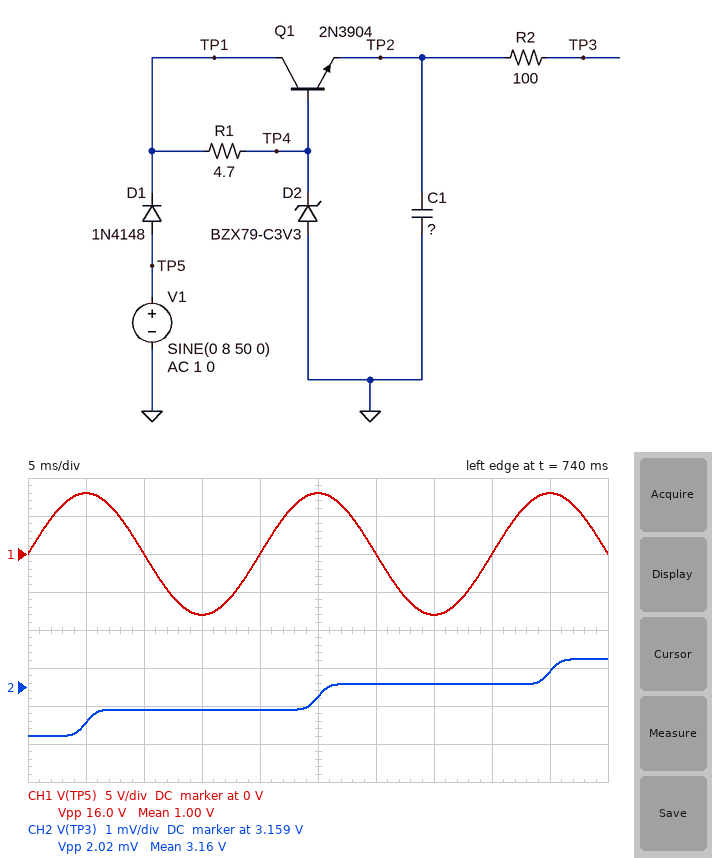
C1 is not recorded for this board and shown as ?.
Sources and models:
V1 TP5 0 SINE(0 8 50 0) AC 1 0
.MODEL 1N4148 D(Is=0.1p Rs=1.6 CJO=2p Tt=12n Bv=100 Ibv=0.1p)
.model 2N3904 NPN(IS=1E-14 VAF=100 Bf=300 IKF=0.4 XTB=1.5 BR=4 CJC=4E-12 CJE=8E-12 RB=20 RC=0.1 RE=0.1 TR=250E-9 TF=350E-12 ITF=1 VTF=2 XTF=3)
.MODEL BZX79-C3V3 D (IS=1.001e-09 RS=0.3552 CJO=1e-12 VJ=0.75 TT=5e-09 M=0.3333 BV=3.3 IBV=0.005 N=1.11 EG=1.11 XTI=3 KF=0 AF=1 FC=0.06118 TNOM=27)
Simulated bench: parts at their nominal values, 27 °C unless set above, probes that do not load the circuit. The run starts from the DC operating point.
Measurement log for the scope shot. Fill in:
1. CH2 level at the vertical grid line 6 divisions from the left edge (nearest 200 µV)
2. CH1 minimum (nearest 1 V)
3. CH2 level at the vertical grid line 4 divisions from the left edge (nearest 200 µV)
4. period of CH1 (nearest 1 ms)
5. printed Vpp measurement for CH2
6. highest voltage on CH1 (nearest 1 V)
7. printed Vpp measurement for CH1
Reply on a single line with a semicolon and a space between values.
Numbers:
3.1590 V; -8 V; 3.1584 V; 20 ms; 2.02 mV; 8 V; 16.0 V
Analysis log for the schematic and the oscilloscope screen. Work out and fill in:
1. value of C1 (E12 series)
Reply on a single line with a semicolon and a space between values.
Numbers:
3.3 µF
